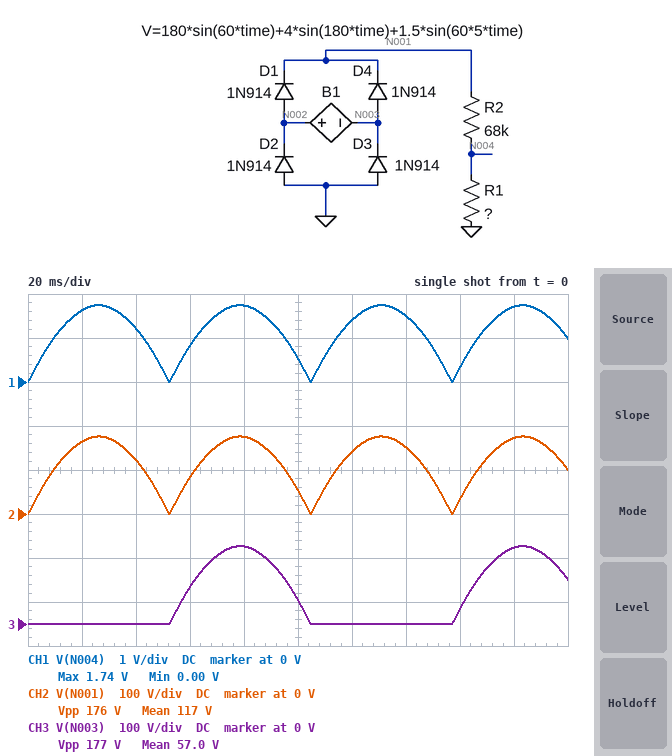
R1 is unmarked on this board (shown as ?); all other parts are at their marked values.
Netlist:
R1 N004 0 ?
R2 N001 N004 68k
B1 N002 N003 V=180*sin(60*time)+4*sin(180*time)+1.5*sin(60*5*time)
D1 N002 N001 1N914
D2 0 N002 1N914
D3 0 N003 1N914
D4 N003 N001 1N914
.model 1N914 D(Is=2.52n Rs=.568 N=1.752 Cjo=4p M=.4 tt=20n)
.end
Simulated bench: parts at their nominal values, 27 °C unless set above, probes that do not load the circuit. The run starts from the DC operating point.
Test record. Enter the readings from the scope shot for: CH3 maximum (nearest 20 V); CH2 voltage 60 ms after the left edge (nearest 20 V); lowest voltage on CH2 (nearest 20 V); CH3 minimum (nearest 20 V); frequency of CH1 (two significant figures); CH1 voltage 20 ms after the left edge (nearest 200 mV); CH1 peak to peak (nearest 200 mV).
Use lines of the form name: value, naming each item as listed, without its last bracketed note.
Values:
CH3 maximum: 180 V
CH2 voltage 60 ms after the left edge: 80 V
lowest voltage on CH2: 0 V
CH3 minimum: 0 V
frequency of CH1: 19 Hz
CH1 voltage 20 ms after the left edge: 1.6 V
CH1 peak to peak: 1.8 V
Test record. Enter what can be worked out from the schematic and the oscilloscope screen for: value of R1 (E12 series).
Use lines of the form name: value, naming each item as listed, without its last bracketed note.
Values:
value of R1: 680 Ω
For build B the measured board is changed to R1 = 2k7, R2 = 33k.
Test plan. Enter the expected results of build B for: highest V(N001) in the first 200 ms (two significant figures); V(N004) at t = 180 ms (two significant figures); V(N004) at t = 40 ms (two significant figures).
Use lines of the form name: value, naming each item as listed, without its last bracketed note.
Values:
highest V(N001) in the first 200 ms: 180 V
V(N004) at t = 180 ms: 13 V
V(N004) at t = 40 ms: 9.3 V
